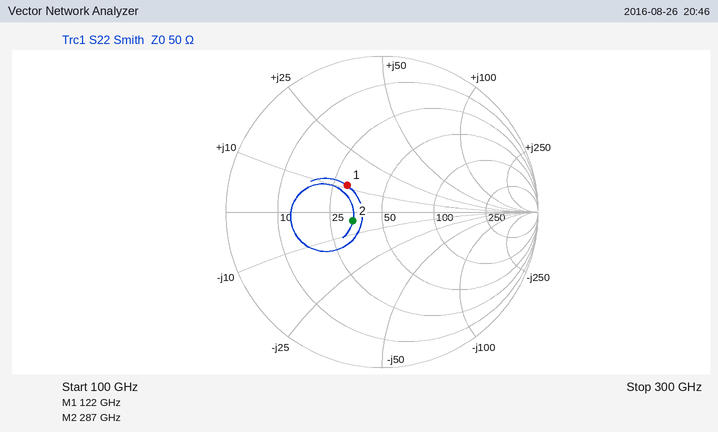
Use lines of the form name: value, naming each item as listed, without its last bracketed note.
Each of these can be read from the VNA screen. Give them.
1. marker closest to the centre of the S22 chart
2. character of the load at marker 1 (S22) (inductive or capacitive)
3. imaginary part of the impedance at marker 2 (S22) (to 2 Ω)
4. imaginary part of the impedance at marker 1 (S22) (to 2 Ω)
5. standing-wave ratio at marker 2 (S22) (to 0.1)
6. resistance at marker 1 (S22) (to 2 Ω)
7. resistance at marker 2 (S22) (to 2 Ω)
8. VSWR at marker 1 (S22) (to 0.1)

marker closest to the centre of the S22 chart: marker 2
character of the load at marker 1 (S22): inductive
imaginary part of the impedance at marker 2 (S22): -4 Ω
imaginary part of the impedance at marker 1 (S22): +12 Ω
standing-wave ratio at marker 2 (S22): 1.5
resistance at marker 1 (S22): 30 Ω
resistance at marker 2 (S22): 34 Ω
VSWR at marker 1 (S22): 1.8
